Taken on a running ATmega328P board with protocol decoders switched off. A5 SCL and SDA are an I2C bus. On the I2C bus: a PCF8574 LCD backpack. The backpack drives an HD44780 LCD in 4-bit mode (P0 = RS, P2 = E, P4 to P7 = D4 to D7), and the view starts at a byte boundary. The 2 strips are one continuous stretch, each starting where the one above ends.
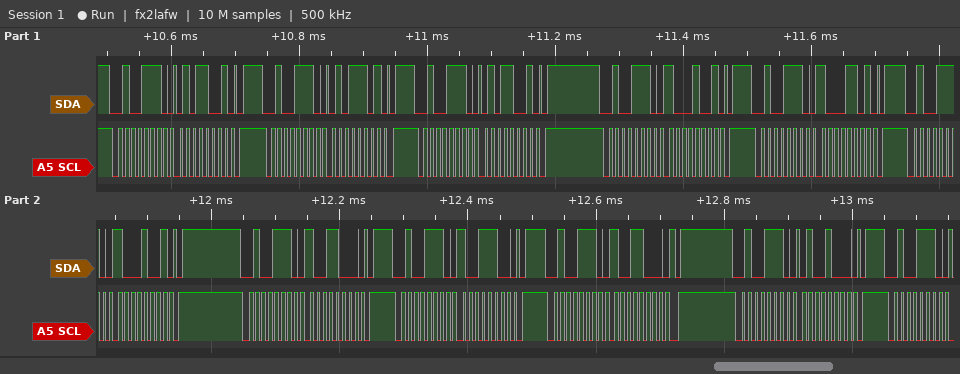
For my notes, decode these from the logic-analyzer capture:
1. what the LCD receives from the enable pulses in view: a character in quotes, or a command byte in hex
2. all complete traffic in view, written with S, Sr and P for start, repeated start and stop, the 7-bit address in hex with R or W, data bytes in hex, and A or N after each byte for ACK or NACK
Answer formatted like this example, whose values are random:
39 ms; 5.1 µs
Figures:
'X'; S 27W A 59 A P S 27W A 5D A P S 27W A 59 A P S 27W A 89 A P S 27W A 8D A P S 27W A 89 A P S 27W A 98 A P S 27W A 9C A P S 27W A 98 A P S 27W A 48 A P S 27W A
